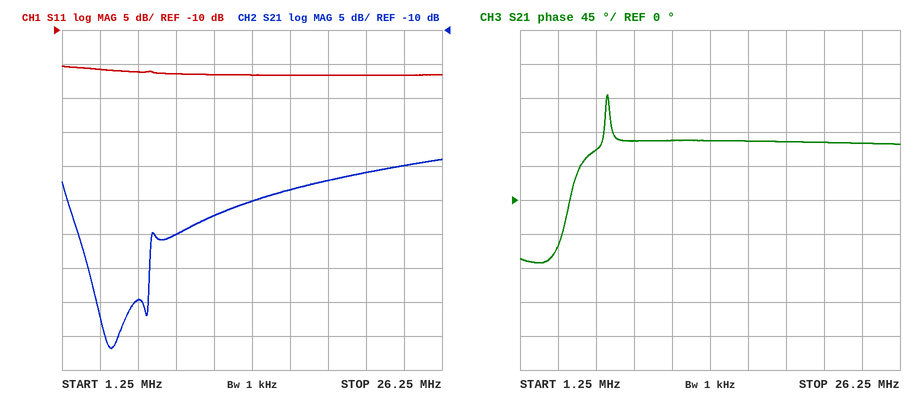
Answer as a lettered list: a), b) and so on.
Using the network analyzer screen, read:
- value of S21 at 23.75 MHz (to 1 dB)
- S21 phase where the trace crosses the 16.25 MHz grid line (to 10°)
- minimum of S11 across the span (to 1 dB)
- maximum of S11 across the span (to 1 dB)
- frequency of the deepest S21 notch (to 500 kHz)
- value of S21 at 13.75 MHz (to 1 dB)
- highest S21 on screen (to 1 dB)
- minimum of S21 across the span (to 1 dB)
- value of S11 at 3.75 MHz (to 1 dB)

a) -30 dB
b) 80°
c) -17 dB
d) -15 dB
e) 4.5 MHz
f) -35 dB
g) -29 dB
h) -57 dB
i) -16 dB
